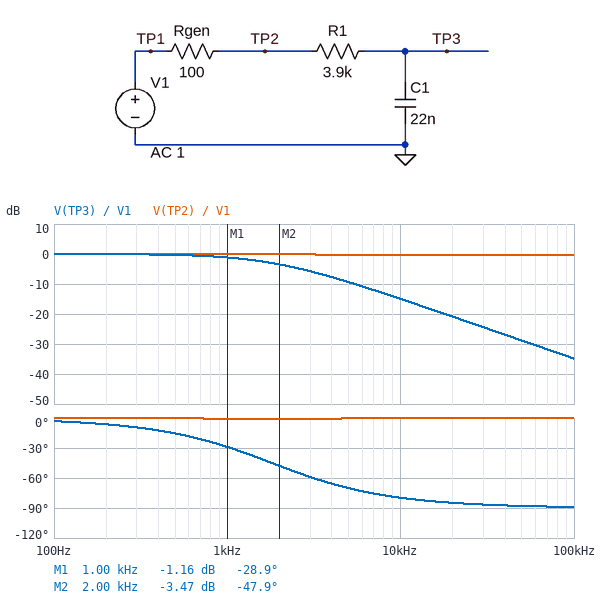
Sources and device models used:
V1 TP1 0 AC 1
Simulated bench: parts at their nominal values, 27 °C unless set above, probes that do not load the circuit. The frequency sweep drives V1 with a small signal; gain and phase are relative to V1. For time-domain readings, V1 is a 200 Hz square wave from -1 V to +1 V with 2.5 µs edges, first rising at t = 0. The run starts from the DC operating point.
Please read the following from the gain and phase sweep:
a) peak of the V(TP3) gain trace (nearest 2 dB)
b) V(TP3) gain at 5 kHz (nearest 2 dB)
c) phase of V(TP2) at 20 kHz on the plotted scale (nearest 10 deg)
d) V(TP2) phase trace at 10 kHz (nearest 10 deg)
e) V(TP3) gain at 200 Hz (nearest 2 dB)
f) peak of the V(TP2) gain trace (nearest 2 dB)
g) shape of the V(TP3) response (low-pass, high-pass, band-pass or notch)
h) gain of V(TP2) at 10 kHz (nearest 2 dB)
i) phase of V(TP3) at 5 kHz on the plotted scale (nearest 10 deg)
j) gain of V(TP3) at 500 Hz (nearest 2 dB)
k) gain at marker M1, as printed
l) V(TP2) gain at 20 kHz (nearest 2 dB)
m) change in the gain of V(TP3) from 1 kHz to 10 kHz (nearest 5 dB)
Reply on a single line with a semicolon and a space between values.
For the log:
0 dB; -10 dB; 0 deg; 0 deg; 0 dB; 0 dB; low-pass; 0 dB; -70 deg; 0 dB; -1.16 dB; 0 dB; -15 dB
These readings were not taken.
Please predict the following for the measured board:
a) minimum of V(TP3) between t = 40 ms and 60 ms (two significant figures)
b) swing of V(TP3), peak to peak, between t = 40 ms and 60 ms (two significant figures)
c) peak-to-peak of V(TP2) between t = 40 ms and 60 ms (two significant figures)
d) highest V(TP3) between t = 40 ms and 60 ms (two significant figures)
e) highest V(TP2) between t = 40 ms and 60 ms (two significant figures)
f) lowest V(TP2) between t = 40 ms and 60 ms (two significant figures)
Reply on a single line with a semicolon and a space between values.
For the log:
-1.0 V; 2.0 V; 2.0 V; 1.0 V; 1.0 V; -1.0 V
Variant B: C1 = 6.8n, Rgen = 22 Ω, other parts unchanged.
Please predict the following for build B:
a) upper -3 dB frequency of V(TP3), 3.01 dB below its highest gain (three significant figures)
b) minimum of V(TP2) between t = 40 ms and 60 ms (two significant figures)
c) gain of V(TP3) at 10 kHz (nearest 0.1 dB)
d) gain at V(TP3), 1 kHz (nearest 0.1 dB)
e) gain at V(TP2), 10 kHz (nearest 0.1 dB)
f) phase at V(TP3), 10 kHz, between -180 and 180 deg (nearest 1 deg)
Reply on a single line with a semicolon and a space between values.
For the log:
5.97 kHz; -1.0 V; -5.8 dB; -0.1 dB; 0 dB; -59 deg
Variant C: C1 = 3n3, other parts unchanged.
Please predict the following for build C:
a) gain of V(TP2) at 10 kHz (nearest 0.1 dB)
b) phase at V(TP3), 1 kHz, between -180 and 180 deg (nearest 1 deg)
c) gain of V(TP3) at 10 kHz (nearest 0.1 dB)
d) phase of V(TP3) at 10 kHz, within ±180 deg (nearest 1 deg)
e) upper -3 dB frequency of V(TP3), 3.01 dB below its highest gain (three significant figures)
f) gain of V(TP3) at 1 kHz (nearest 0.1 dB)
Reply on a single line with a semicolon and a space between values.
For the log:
-0.1 dB; -5 deg; -2.3 dB; -40 deg; 12.1 kHz; 0 dB
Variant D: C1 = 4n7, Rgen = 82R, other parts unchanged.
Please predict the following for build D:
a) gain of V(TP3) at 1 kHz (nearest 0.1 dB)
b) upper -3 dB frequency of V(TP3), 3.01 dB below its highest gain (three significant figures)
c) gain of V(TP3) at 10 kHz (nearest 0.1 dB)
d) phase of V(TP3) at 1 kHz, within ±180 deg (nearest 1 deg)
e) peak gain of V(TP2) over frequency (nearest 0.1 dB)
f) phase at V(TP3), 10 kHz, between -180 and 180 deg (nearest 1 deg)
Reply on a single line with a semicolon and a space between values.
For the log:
-0.1 dB; 8.50 kHz; -3.8 dB; -7 deg; 0 dB; -50 deg
